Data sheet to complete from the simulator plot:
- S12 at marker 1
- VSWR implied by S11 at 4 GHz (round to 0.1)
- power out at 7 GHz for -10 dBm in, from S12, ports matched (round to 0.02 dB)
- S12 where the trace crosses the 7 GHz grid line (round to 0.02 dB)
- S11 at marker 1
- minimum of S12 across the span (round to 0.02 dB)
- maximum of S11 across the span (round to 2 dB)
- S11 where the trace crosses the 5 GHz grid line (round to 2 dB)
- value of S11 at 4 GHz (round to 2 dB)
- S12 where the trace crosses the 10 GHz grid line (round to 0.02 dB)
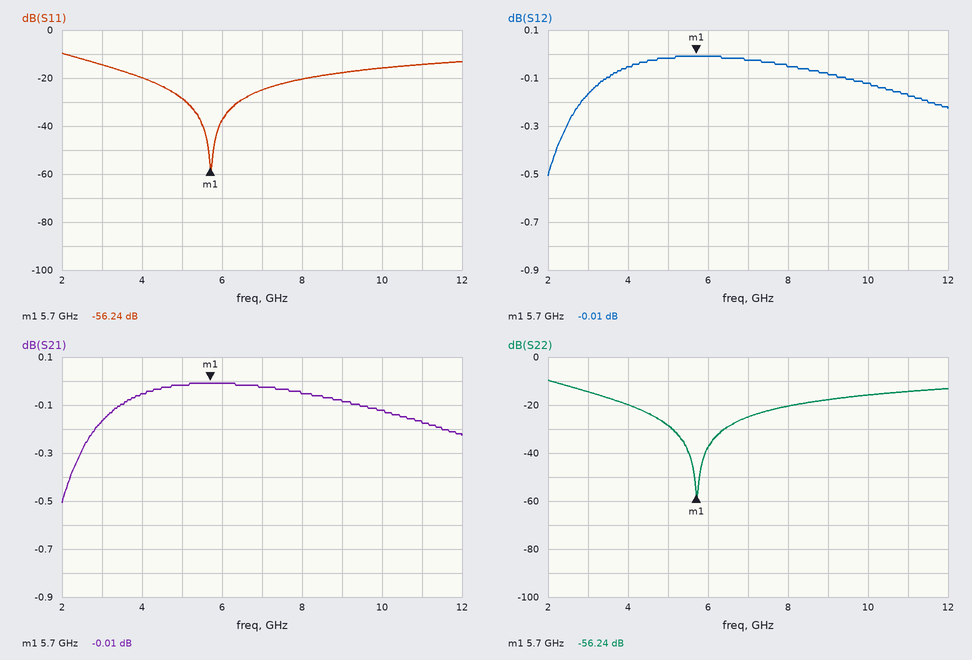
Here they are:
-0.01 dB
1.2
-10.02 dBm
-0.02 dB
-56.24 dB
-0.50 dB
-10 dB
-28 dB
-20 dB
-0.12 dB
